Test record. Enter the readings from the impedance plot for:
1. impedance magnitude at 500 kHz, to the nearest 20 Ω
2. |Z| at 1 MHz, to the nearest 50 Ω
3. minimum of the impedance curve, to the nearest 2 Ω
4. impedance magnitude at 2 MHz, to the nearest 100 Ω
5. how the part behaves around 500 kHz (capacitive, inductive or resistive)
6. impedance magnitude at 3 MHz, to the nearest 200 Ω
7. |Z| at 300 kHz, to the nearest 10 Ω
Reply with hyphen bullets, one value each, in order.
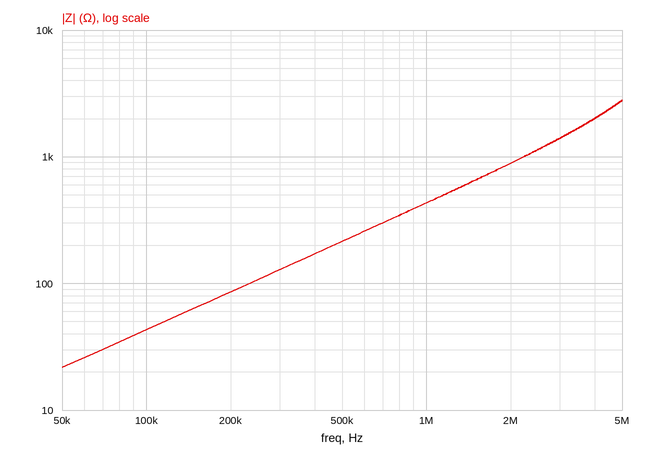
- 220 Ω
- 450 Ω
- 22 Ω
- 900 Ω
- inductive
- 1.4 kΩ
- 130 Ω
